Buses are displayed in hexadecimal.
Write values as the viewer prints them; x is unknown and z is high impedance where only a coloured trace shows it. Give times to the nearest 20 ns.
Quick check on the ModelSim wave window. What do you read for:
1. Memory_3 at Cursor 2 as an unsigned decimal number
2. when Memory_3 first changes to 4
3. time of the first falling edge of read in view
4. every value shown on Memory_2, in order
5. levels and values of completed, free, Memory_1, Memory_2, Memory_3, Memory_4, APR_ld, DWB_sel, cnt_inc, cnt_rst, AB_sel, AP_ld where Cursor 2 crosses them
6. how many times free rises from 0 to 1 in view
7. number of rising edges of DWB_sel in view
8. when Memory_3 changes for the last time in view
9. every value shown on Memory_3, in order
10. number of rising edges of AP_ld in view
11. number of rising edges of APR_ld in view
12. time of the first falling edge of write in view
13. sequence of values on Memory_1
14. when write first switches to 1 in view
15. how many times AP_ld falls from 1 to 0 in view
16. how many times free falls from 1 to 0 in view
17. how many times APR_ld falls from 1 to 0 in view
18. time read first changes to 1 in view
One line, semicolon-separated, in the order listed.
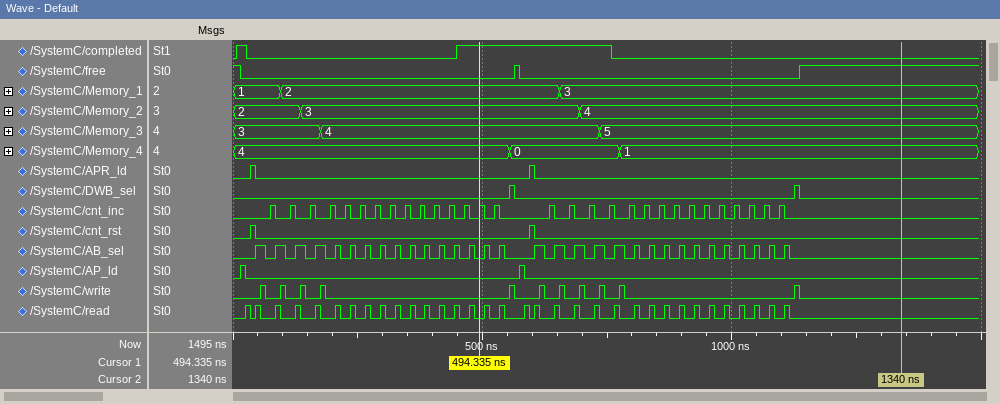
5; 180 ns; 40 ns; 2, 3, 4; completed=0, free=1, Memory_1=3, Memory_2=4, Memory_3=5, Memory_4=1, APR_ld=0, DWB_sel=0, cnt_inc=0, cnt_rst=0, AB_sel=0, AP_ld=0; 2; 2; 740 ns; 3, 4, 5; 2; 2; 60 ns; 1, 2, 3; 60 ns; 2; 2; 2; 20 ns
